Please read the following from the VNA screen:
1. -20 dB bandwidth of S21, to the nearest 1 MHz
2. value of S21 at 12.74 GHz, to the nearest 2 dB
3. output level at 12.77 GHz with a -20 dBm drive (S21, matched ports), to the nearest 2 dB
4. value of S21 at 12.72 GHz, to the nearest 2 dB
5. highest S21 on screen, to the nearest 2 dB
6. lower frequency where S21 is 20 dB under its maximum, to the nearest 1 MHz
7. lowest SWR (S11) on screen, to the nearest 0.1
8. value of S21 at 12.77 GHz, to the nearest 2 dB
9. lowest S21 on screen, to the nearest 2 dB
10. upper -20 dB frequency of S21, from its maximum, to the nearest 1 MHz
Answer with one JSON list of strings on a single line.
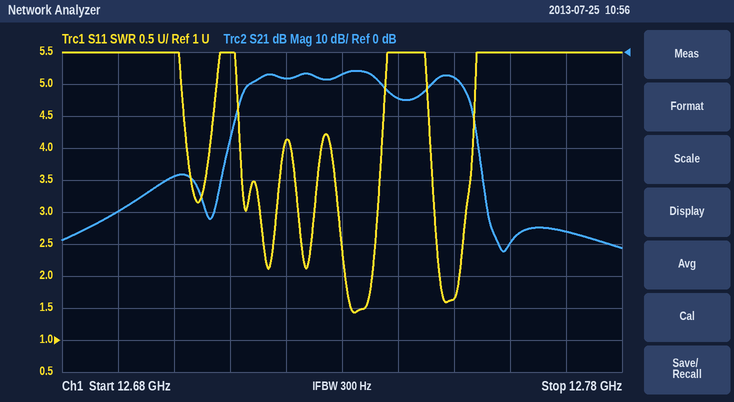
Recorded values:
["44 MHz", "-14 dB", "-76 dBm", "-8 dB", "-6 dB", "12.710 GHz", "1.4", "-56 dB", "-62 dB", "12.754 GHz"]
